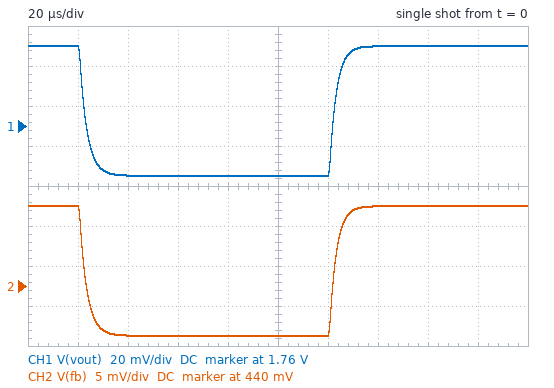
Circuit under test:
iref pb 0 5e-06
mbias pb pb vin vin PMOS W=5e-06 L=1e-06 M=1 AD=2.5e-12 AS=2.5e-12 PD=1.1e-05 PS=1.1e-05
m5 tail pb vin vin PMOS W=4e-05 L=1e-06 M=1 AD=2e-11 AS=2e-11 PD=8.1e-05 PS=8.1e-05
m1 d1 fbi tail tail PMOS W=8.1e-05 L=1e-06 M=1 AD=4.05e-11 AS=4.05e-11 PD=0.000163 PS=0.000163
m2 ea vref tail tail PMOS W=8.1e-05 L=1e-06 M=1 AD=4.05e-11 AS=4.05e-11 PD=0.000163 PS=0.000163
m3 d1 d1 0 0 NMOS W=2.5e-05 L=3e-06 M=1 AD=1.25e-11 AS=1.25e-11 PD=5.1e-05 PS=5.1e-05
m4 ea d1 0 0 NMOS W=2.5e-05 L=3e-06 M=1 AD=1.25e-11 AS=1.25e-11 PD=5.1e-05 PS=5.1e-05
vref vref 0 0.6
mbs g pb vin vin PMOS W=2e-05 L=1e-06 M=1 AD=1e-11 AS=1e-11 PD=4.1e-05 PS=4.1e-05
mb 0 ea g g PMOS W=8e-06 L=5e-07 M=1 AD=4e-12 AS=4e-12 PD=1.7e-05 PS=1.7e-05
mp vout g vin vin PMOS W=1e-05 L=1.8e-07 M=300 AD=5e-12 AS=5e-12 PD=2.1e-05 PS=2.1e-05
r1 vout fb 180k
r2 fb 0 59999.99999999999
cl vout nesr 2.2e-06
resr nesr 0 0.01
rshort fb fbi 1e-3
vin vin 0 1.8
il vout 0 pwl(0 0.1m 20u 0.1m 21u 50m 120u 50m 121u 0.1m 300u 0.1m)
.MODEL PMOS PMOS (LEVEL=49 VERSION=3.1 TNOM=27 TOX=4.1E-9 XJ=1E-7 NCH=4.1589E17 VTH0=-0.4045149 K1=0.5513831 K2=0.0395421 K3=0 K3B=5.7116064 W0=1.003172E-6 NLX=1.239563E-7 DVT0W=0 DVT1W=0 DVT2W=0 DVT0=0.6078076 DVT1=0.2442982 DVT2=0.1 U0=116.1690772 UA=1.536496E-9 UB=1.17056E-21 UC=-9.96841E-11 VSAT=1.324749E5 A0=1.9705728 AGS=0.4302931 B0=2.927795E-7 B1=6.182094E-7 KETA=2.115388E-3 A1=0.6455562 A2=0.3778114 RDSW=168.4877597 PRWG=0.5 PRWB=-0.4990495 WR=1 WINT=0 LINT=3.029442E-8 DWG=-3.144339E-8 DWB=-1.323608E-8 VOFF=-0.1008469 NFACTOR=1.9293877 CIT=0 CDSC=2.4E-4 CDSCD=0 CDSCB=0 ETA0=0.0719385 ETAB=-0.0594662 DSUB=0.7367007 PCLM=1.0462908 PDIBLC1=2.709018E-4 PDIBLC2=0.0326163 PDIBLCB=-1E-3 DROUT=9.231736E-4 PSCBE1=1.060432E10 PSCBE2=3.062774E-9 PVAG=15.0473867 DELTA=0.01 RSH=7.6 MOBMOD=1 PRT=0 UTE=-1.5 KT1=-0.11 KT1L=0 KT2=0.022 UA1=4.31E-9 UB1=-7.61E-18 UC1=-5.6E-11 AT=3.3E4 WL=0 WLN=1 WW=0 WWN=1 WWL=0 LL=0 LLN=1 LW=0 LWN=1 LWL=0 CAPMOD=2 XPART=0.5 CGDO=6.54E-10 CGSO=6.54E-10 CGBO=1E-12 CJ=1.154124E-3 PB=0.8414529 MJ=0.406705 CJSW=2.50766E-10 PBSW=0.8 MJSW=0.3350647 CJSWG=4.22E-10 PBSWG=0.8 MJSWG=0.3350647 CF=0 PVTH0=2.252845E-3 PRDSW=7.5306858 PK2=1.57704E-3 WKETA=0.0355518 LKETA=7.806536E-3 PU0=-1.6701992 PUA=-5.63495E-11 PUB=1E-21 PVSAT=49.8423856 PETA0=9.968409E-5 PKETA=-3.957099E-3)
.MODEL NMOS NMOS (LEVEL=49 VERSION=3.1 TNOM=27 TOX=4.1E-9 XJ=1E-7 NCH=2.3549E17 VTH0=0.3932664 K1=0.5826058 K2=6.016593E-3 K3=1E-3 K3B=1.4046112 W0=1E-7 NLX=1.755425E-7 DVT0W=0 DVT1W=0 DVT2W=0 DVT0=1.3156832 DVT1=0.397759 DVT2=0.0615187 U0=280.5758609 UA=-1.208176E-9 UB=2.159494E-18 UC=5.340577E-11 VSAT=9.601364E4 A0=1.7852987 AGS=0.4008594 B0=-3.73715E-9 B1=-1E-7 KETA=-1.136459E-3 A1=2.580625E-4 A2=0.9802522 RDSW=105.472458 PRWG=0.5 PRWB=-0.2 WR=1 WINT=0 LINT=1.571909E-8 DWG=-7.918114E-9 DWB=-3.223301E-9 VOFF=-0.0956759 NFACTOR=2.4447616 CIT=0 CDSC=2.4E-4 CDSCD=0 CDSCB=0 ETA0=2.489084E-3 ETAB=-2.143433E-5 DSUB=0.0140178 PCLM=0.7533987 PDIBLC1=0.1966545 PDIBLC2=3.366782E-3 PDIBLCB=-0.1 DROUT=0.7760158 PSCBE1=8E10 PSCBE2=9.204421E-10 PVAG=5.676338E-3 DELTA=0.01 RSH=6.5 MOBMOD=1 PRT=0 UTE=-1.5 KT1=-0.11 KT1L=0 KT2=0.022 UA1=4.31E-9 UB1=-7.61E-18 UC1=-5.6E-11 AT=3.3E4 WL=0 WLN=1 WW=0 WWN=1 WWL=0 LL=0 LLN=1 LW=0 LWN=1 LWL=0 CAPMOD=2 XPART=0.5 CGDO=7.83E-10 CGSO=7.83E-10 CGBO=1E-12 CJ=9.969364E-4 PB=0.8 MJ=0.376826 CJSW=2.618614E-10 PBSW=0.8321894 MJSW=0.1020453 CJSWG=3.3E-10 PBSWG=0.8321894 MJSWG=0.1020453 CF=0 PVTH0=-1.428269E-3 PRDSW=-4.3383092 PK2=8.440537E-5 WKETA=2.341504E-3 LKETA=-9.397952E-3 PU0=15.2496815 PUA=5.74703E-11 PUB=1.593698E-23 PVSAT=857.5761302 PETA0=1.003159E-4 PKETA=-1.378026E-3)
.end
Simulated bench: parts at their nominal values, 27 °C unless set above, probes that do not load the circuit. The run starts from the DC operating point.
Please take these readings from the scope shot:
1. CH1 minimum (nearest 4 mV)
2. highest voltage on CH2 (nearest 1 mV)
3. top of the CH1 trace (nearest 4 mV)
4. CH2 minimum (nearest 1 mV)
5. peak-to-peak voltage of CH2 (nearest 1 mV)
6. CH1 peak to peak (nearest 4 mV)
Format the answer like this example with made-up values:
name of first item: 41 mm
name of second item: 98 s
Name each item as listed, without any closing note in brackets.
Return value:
CH1 minimum: 1.736 V
highest voltage on CH2: 450 mV
top of the CH1 trace: 1.800 V
CH2 minimum: 434 mV
peak-to-peak voltage of CH2: 16 mV
CH1 peak to peak: 64 mV
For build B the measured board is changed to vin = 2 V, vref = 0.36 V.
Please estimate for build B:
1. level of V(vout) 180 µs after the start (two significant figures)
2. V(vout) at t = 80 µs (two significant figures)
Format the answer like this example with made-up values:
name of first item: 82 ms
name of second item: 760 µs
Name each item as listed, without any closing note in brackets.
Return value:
level of V(vout) 180 µs after the start: 1.5 V
V(vout) at t = 80 µs: 1.4 V
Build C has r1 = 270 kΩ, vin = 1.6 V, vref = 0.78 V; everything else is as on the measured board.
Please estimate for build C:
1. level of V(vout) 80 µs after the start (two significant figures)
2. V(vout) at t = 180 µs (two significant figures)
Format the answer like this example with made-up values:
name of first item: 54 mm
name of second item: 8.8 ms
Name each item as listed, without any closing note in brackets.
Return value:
level of V(vout) 80 µs after the start: 1.5 V
V(vout) at t = 180 µs: 1.6 V
